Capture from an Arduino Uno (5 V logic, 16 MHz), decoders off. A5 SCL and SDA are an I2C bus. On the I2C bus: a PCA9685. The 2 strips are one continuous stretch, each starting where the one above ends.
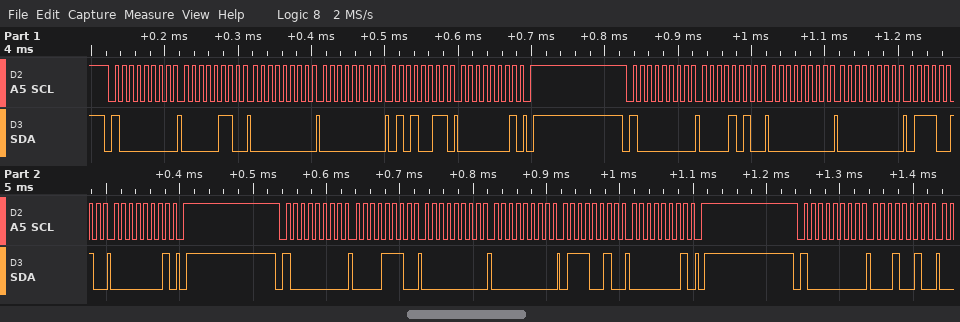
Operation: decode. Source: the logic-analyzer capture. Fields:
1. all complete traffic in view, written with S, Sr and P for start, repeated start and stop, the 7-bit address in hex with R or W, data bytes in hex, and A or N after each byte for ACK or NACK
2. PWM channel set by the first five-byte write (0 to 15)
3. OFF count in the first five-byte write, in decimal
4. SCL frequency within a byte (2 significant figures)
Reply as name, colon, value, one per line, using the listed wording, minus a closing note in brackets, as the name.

all complete traffic in view, written with S, Sr and P for start, repeated start and stop, the 7-bit address in hex with R or W, data bytes in hex, and A or N after each byte for ACK or NACK: S 40W A 06 A 00 A 00 A 53 A 01 A P S 40W A 0A A 00 A 00 A 72 A 01 A P S 40W A 0E A 00 A 00 A 72 A 01 A P S 40W A 12 A
PWM channel set by the first five-byte write: 0
OFF count in the first five-byte write, in decimal: 339
SCL frequency within a byte: 100 kHz
